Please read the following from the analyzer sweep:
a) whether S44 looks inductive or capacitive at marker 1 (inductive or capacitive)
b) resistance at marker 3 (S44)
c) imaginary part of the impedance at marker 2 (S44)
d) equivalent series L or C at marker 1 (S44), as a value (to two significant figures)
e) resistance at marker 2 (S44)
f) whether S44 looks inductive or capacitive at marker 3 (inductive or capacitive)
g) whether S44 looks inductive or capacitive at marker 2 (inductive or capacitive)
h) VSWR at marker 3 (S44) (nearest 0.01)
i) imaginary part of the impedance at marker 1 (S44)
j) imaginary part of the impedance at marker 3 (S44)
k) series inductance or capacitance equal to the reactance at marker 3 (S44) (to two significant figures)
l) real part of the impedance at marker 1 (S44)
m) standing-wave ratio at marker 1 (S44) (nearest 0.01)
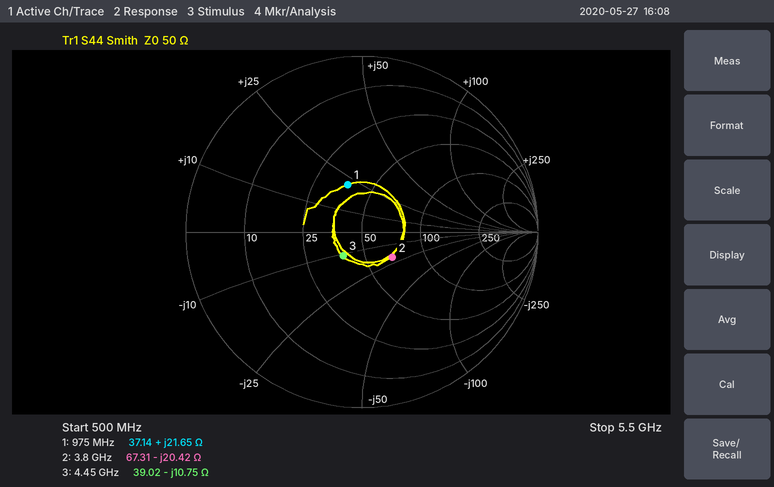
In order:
inductive
39.02 Ω
-20.42 Ω
3.5 nH
67.31 Ω
capacitive
capacitive
1.41
+21.65 Ω
-10.75 Ω
3.3 pF
37.14 Ω
1.78
